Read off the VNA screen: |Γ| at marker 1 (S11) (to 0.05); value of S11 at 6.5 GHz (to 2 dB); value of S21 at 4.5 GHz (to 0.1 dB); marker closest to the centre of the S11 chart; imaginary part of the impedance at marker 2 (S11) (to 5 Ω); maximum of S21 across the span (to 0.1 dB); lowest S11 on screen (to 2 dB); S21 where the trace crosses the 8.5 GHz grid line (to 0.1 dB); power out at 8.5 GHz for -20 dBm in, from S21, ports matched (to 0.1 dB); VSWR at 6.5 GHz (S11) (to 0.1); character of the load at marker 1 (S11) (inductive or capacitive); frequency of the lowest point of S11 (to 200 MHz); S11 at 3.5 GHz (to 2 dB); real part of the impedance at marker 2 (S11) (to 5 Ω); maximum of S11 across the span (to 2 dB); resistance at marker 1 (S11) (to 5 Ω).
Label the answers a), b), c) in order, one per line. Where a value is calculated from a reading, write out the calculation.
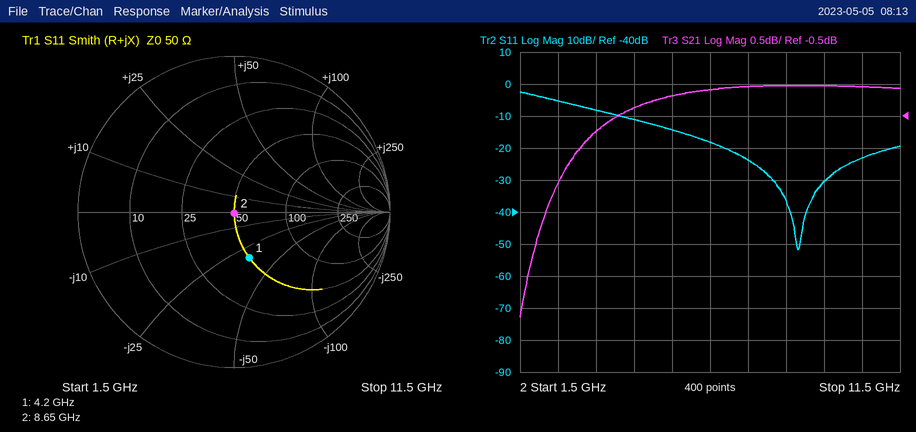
a) 0.30
b) -18 dB
c) -0.4 dB
d) marker 2
e) 0 Ω
f) 0.0 dB
g) -52 dB
h) 0.0 dB
i) -20 dBm + (0.0 dB) = -20.0 dBm
j) |Γ| = 10^(-18/20) = 0.1259; VSWR = (1 + 0.1259)/(1 − 0.1259) ≈ 1.3
k) capacitive
l) 8.8 GHz
m) -8 dB
n) 50 Ω
o) -2 dB
p) 50 Ω
